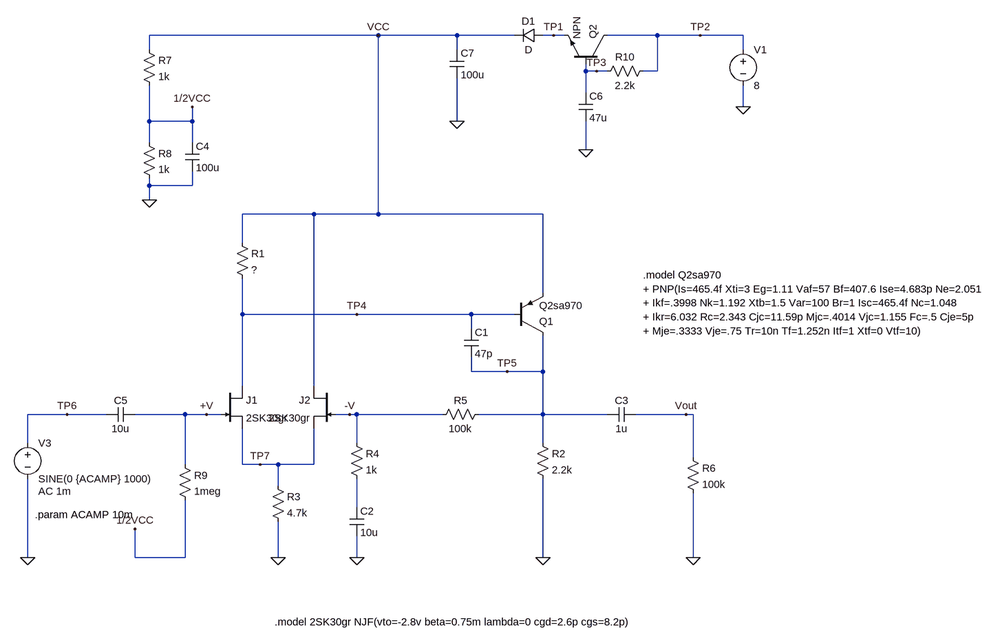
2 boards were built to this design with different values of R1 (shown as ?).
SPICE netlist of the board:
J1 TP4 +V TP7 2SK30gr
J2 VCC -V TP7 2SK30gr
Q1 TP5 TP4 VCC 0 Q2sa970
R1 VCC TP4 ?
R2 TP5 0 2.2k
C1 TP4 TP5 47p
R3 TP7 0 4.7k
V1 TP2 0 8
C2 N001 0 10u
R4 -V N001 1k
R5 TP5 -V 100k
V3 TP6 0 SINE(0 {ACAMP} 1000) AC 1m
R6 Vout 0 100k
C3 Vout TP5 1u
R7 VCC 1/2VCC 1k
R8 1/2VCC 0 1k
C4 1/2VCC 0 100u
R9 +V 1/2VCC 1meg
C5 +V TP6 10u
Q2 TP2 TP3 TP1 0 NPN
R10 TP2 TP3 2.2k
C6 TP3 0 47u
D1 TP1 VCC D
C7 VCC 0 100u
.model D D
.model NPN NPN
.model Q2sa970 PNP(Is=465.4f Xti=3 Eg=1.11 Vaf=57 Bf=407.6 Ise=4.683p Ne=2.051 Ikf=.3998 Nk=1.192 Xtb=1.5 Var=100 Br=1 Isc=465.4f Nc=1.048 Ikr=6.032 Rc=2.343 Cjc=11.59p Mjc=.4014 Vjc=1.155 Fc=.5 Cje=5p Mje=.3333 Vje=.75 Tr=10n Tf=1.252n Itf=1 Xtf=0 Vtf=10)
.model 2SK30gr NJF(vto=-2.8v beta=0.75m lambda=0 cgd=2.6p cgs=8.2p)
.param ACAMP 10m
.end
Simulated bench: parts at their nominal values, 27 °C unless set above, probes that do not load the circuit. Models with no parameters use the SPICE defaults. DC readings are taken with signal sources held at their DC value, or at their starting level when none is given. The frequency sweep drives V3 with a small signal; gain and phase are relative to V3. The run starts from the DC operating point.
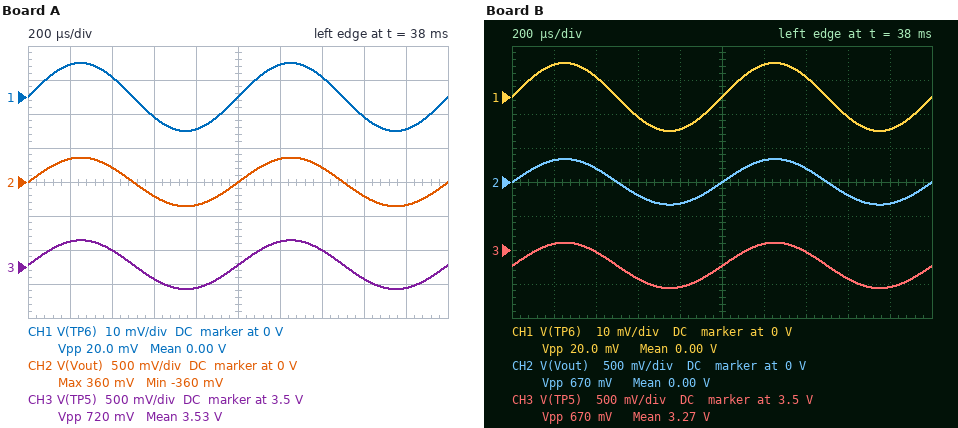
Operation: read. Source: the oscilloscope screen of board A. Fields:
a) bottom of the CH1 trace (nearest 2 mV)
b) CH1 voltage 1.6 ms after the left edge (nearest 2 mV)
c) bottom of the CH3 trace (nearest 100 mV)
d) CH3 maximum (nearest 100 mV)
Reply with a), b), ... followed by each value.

a) -10 mV
b) -6 mV
c) 3.2 V
d) 3.9 V
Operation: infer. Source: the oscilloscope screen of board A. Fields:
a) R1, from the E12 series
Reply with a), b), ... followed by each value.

a) 1.8 kΩ
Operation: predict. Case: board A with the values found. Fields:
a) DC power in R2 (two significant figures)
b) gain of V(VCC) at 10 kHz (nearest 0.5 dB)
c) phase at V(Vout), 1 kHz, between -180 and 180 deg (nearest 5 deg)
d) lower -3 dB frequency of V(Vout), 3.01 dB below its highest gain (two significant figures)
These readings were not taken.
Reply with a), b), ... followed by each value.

a) 5.7 mW
b) -51.5 dB
c) 0 deg
d) 8.1 Hz
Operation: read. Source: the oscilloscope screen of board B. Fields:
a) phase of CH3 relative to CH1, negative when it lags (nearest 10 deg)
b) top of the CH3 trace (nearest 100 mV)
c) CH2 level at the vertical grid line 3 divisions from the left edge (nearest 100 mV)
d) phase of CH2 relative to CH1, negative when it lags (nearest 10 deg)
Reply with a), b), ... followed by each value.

a) 0 deg
b) 3.6 V
c) -200 mV
d) 0 deg
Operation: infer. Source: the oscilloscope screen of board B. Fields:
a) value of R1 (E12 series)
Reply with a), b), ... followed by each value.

a) 1.2 kΩ
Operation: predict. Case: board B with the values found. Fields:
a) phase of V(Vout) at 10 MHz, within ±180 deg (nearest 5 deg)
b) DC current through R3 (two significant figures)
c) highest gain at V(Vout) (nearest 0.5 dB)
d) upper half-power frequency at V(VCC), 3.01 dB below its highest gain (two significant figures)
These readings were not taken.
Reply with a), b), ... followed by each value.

a) -120 deg
b) 1.1 mA
c) 30.5 dB
d) 200 Hz
